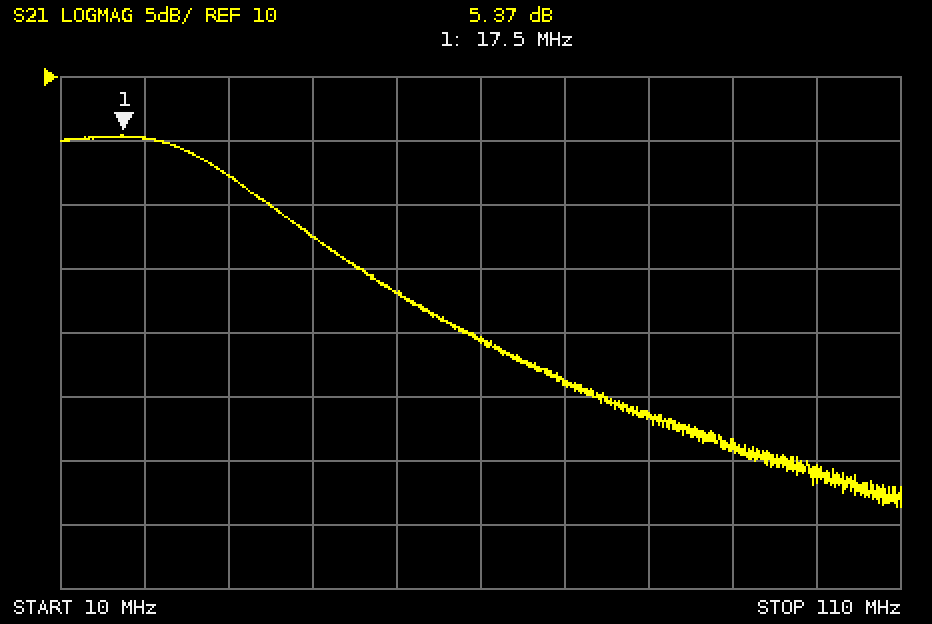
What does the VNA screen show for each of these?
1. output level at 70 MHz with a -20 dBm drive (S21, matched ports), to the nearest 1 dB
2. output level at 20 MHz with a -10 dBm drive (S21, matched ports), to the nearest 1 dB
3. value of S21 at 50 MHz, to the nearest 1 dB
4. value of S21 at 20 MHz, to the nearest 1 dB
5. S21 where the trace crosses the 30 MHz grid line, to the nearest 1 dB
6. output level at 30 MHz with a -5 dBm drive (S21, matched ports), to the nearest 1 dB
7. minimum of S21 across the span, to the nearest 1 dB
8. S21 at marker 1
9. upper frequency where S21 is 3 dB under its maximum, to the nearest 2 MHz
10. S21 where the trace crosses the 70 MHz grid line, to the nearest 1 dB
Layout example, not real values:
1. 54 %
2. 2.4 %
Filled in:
1. -34 dBm
2. -5 dBm
3. -7 dB
4. 5 dB
5. 2 dB
6. -3 dBm
7. -24 dB
8. 5.37 dB
9. 30 MHz
10. -14 dB
